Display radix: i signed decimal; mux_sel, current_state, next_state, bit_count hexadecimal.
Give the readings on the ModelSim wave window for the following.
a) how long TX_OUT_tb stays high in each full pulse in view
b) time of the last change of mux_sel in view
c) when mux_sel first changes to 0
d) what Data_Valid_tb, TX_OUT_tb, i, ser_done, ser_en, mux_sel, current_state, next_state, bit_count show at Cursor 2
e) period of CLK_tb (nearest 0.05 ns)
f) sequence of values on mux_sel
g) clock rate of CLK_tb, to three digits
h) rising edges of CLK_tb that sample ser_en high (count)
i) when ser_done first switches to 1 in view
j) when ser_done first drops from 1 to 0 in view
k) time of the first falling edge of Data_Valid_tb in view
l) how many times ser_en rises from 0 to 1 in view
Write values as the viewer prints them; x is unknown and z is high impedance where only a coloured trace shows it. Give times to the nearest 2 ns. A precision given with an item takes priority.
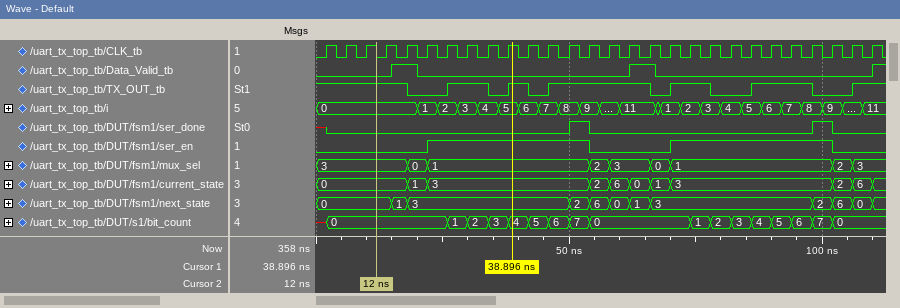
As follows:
8 ns, 4 ns, 20 ns, 8 ns, 12 ns
106 ns
18 ns
Data_Valid_tb=0, TX_OUT_tb=1, i=0, ser_done=0, ser_en=0, mux_sel=3, current_state=0, next_state=0, bit_count=0
4 ns
3, 0, 1, 2, 3, 0, 1, 2, 3
250 MHz
16
50 ns
54 ns
20 ns
2
